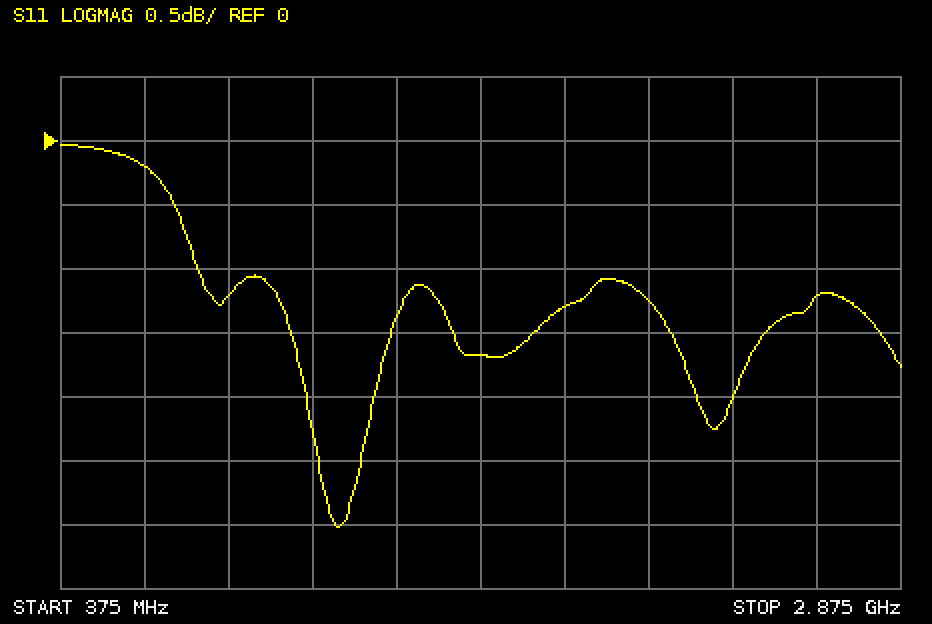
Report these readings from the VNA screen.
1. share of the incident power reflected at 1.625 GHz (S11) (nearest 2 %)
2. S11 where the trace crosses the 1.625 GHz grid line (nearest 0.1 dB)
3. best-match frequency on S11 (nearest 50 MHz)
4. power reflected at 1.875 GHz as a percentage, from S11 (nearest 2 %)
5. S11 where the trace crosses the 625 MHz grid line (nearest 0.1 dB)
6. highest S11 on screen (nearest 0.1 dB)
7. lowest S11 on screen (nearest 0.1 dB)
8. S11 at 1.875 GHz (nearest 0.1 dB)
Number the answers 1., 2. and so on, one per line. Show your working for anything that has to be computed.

1. 10^(-1.7/10) ≈ 68 %
2. -1.7 dB
3. 1.20 GHz
4. 10^(-1.3/10) ≈ 74 %
5. -0.2 dB
6. 0.0 dB
7. -3.0 dB
8. -1.3 dB
